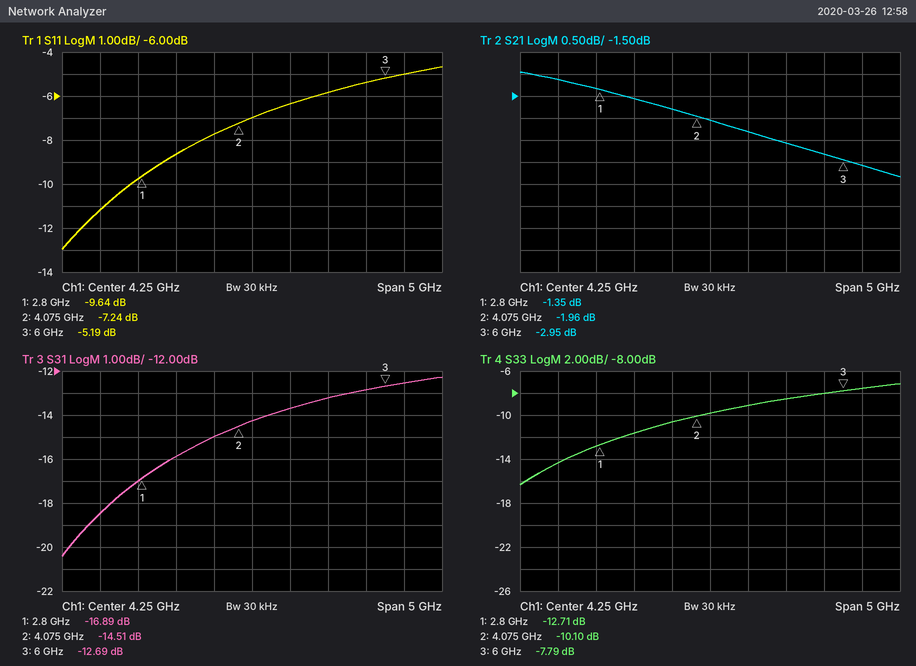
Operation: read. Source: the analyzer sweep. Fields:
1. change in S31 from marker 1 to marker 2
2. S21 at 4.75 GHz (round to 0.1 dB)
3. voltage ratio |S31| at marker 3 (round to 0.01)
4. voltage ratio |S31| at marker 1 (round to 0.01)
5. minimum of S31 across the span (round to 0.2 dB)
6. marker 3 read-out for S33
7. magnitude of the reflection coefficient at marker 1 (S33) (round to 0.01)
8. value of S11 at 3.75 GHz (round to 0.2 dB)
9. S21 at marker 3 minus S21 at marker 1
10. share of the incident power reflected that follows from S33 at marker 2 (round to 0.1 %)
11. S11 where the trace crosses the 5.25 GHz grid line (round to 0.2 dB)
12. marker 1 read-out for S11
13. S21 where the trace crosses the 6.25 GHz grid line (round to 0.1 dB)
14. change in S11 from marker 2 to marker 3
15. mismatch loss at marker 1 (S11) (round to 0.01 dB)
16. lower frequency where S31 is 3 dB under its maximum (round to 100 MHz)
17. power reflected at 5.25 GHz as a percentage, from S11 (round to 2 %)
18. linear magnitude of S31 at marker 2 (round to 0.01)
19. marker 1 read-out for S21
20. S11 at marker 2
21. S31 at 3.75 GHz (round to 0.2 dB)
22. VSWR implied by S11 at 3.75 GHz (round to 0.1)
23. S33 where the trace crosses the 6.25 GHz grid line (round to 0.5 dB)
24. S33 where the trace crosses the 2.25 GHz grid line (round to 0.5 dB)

2.38 dB
-2.3 dB
0.23
0.14
-20.4 dB
-7.79 dB
0.23
-7.8 dB
-1.60 dB
9.8 %
-5.8 dB
-9.64 dB
-3.1 dB
2.05 dB
0.50 dB
3.6 GHz
26 %
0.19
-1.35 dB
-7.24 dB
-15.0 dB
2.4
-7.5 dB
-14.5 dB
